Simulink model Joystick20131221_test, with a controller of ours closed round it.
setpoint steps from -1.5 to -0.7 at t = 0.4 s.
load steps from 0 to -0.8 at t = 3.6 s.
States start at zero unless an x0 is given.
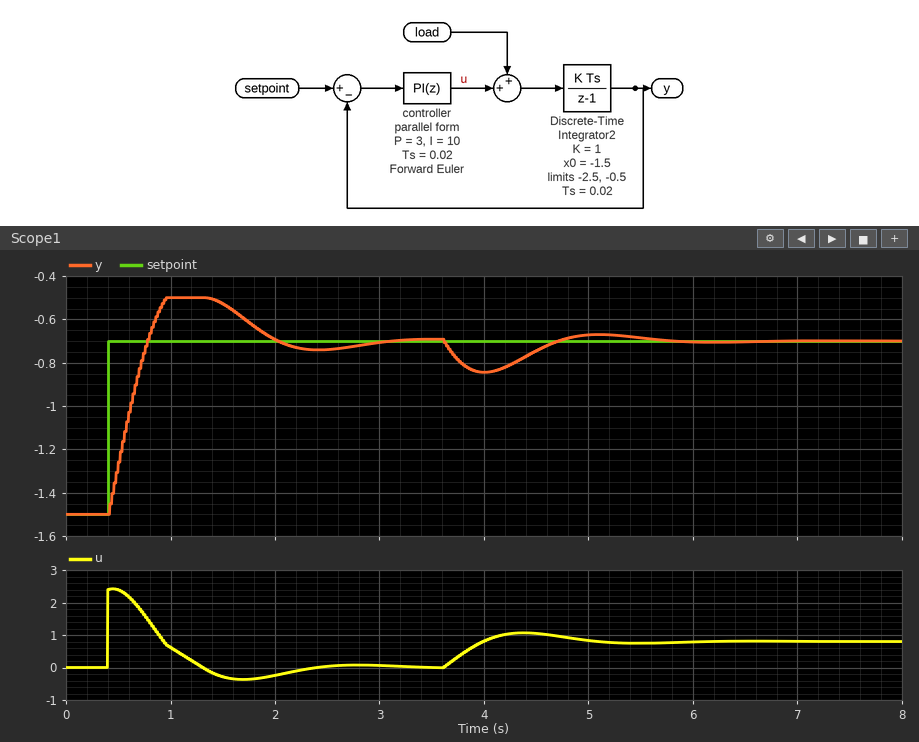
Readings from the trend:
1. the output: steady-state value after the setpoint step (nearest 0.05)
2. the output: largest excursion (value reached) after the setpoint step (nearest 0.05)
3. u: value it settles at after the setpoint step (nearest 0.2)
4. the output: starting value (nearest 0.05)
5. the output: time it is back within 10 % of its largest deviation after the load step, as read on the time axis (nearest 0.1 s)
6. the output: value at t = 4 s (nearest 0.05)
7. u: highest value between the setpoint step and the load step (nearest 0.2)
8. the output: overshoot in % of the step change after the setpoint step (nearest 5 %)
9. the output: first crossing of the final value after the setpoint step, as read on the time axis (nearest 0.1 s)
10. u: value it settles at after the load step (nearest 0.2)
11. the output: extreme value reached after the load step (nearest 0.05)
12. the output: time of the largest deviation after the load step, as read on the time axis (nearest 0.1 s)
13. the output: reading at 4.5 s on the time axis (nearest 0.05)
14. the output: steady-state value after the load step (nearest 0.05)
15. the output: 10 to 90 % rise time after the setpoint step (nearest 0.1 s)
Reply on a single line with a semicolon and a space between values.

-0.70; -0.50; 0.0; -1.50; 5.5 s; -0.85; 2.4; 25 %; 0.8 s; 0.8; -0.85; 4.0 s; -0.75; -0.70; 0.3 s
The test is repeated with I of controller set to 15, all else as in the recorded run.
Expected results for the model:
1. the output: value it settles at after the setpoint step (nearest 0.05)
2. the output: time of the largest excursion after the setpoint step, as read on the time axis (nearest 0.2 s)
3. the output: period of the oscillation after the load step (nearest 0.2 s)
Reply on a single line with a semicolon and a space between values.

-0.70; 0.8 s; 1.8 s
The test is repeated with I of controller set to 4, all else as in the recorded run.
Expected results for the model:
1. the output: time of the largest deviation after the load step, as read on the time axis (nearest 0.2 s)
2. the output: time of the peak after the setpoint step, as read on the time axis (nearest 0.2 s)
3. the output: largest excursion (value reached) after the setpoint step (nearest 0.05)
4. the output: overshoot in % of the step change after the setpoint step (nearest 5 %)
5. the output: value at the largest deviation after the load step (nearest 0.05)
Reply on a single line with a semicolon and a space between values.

4.2 s; 1.4 s; -0.55; 20 %; -0.90
